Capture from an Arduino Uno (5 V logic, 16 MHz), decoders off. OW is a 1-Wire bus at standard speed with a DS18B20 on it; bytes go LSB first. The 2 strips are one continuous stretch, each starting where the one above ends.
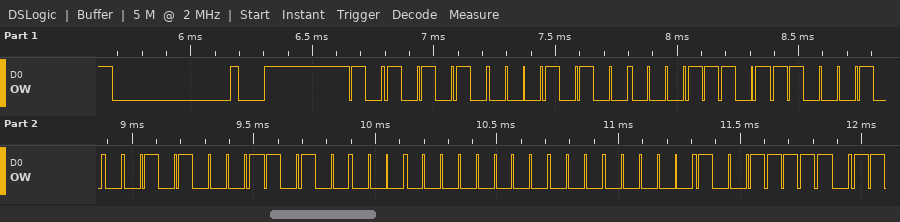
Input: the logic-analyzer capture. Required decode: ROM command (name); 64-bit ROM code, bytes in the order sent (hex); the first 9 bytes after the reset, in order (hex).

Match ROM
28 B8 23 8A 05 00 00 F9
55 28 B8 23 8A 05 00 00 F9
